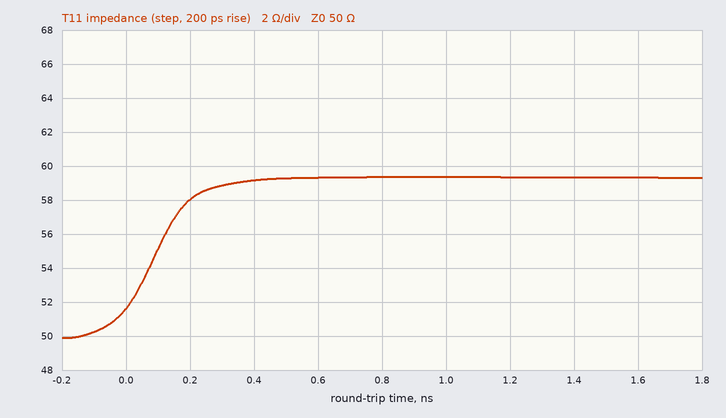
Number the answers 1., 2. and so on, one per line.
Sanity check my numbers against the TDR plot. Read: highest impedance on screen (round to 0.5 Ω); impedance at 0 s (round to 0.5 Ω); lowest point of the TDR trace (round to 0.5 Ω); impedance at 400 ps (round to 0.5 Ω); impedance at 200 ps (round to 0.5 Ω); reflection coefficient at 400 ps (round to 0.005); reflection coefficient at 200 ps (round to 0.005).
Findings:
1. 59.5 Ω
2. 51.5 Ω
3. 50.0 Ω
4. 59.0 Ω
5. 58.0 Ω
6. +0.085
7. +0.075
